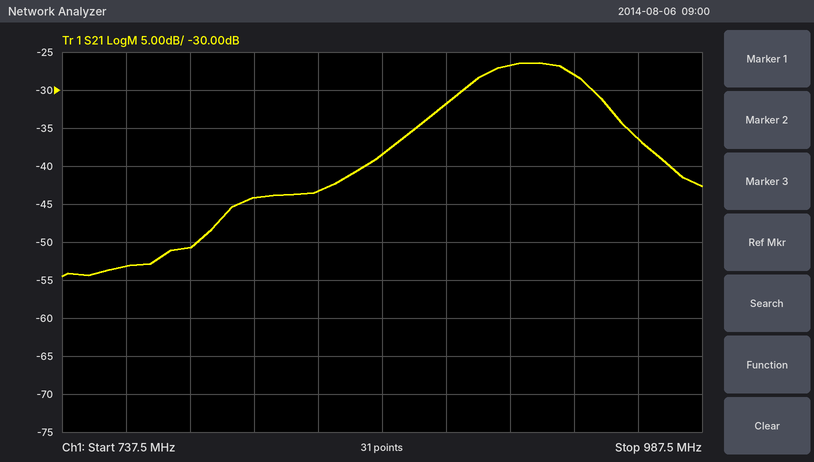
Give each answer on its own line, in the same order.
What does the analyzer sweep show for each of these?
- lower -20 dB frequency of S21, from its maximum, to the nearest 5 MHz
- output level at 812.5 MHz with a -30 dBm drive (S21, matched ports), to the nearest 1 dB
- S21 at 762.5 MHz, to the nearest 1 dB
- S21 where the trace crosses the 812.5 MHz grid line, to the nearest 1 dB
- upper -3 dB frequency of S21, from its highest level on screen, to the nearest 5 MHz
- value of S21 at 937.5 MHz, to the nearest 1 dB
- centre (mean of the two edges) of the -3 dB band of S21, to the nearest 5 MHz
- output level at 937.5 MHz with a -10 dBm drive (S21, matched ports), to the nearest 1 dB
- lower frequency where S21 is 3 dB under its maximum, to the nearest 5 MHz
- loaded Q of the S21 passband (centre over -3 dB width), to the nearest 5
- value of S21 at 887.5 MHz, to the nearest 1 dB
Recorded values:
800 MHz
-74 dBm
-53 dB
-44 dB
945 MHz
-28 dB
920 MHz
-38 dBm
895 MHz
20
-32 dB
